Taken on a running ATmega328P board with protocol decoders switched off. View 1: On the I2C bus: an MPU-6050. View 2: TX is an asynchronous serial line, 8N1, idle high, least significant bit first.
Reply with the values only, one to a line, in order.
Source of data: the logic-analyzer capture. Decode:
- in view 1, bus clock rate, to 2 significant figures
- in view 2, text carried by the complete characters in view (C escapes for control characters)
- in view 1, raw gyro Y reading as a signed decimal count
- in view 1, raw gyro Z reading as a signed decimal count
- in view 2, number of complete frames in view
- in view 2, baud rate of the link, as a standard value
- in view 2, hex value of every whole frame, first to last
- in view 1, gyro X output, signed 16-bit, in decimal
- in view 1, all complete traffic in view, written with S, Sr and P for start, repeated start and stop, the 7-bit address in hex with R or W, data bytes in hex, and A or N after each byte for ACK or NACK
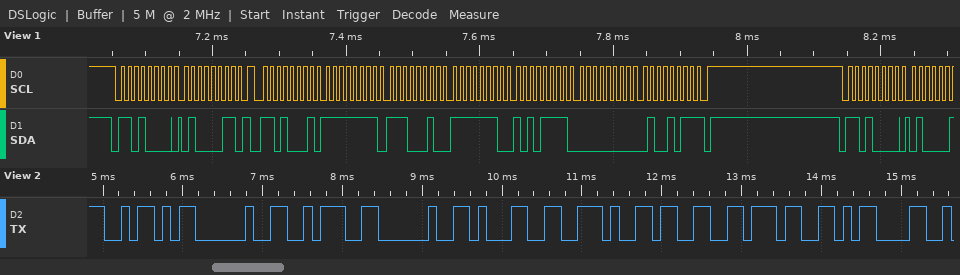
100 kHz
"Z : 1.37\r"
-337
75
9
9600 baud
5A 20 3A 20 31 2E 33 37 0D
-30
S 68W A 43 A Sr 68R A FF A E2 A FE A AF A 00 A 4B N P S 68W A
